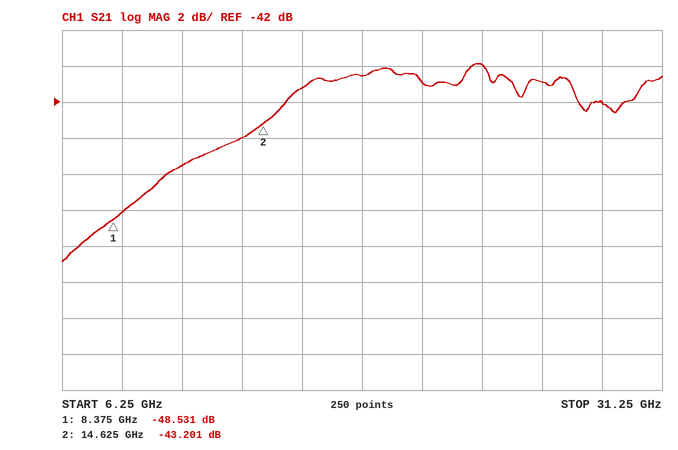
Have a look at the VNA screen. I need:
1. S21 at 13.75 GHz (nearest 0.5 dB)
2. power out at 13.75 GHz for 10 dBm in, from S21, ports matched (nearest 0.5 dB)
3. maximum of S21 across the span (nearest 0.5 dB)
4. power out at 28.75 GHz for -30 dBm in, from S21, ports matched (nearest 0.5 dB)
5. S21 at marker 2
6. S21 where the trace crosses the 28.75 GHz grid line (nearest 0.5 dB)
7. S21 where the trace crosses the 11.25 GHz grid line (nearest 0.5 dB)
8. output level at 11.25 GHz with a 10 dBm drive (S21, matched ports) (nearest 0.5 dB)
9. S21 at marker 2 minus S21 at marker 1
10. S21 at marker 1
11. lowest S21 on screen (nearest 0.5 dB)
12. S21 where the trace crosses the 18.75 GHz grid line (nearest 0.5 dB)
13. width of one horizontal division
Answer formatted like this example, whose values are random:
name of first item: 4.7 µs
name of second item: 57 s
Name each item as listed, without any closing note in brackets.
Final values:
S21 at 13.75 GHz: -44.0 dB
power out at 13.75 GHz for 10 dBm in, from S21, ports matched: -34.0 dBm
maximum of S21 across the span: -40.0 dB
power out at 28.75 GHz for -30 dBm in, from S21, ports matched: -72.0 dBm
S21 at marker 2: -43.201 dB
S21 where the trace crosses the 28.75 GHz grid line: -42.0 dB
S21 where the trace crosses the 11.25 GHz grid line: -45.5 dB
output level at 11.25 GHz with a 10 dBm drive (S21, matched ports): -35.5 dBm
S21 at marker 2 minus S21 at marker 1: 5.330 dB
S21 at marker 1: -48.531 dB
lowest S21 on screen: -51.0 dB
S21 where the trace crosses the 18.75 GHz grid line: -40.5 dB
width of one horizontal division: 2.5 GHz
